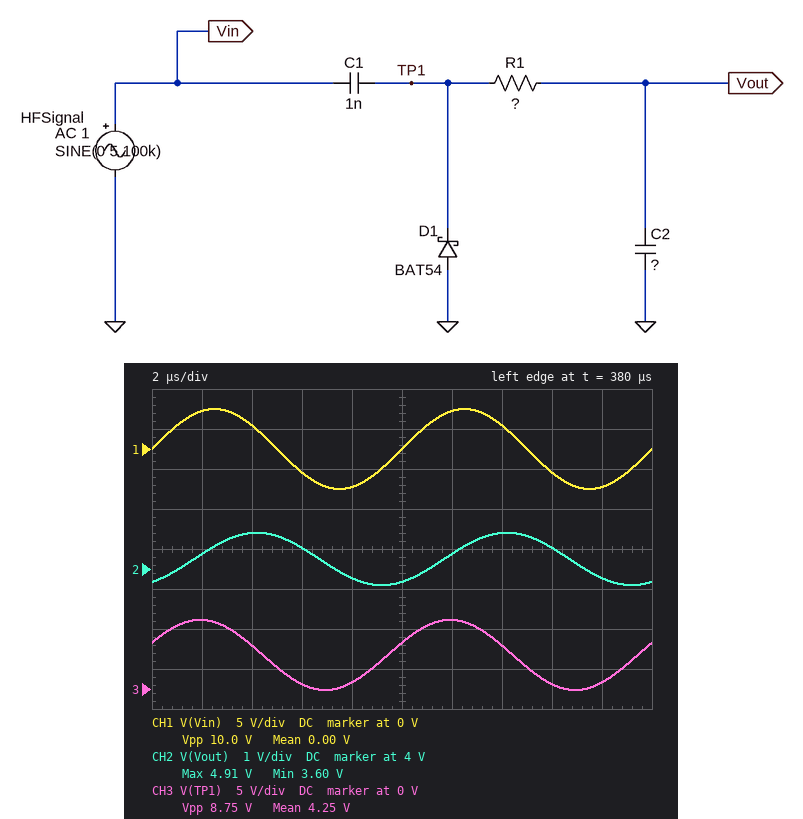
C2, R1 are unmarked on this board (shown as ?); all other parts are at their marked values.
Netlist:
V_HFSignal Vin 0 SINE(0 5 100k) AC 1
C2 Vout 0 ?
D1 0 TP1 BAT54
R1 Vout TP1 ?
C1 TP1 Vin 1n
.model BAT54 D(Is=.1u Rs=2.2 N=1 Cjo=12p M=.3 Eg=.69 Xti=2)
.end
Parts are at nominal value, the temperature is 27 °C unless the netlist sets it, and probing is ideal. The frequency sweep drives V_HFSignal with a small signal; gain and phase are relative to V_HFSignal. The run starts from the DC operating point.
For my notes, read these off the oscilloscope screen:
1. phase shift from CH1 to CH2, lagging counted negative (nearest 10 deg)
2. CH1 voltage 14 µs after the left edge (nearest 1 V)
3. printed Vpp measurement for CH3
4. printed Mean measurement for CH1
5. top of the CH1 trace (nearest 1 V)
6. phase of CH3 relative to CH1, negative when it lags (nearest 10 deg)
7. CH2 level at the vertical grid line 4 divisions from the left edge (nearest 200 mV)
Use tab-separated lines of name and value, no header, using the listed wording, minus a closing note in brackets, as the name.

phase shift from CH1 to CH2, lagging counted negative	-60 deg
CH1 voltage 14 µs after the left edge	3 V
printed Vpp measurement for CH3	8.75 V
printed Mean measurement for CH1	0.00 V
top of the CH1 trace	5 V
phase of CH3 relative to CH1, negative when it lags	20 deg
CH2 level at the vertical grid line 4 divisions from the left edge	3.8 V
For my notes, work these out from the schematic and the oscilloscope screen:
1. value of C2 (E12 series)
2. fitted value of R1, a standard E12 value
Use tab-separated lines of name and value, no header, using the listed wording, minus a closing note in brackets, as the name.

value of C2	2.7 nF
fitted value of R1, a standard E12 value	3.9 kΩ
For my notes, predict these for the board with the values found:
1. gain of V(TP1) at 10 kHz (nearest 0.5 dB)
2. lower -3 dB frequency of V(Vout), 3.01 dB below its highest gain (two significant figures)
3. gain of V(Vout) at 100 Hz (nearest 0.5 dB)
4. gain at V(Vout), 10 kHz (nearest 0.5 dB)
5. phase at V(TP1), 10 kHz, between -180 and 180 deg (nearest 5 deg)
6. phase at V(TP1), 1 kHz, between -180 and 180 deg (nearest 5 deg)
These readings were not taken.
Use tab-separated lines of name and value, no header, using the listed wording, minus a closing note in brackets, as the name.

gain of V(TP1) at 10 kHz	-10.0 dB
lower -3 dB frequency of V(Vout), 3.01 dB below its highest gain	160 Hz
gain of V(Vout) at 100 Hz	-17.0 dB
gain at V(Vout), 10 kHz	-11.5 dB
phase at V(TP1), 10 kHz, between -180 and 180 deg	25 deg
phase at V(TP1), 1 kHz, between -180 and 180 deg	10 deg
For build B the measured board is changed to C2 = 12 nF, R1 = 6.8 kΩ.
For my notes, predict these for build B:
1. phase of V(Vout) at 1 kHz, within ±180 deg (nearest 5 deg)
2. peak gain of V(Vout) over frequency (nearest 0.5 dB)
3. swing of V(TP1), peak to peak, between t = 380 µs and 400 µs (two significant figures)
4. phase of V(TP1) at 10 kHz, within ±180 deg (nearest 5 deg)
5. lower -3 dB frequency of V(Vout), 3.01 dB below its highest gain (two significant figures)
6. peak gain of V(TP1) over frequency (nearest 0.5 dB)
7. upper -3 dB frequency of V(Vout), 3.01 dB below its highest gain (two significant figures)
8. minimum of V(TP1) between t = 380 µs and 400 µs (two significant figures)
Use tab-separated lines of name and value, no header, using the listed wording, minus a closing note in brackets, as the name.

phase of V(Vout) at 1 kHz, within ±180 deg	0 deg
peak gain of V(Vout) over frequency	-22.5 dB
swing of V(TP1), peak to peak, between t = 380 µs and 400 µs	9.5 V
phase of V(TP1) at 10 kHz, within ±180 deg	60 deg
lower -3 dB frequency of V(Vout), 3.01 dB below its highest gain	46 Hz
peak gain of V(TP1) over frequency	0 dB
upper -3 dB frequency of V(Vout), 3.01 dB below its highest gain	26 kHz
minimum of V(TP1) between t = 380 µs and 400 µs	-230 mV
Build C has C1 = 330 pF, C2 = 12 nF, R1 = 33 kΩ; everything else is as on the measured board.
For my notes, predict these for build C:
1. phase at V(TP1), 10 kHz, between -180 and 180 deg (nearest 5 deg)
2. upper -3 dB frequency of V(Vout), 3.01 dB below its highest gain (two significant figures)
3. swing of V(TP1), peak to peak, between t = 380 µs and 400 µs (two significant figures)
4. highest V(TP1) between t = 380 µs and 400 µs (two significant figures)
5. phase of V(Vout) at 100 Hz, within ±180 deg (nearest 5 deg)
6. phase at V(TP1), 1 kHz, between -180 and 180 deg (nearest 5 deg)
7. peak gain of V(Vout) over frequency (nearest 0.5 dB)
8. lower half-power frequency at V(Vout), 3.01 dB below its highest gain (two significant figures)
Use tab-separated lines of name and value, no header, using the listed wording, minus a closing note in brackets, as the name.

phase at V(TP1), 10 kHz, between -180 and 180 deg	55 deg
upper -3 dB frequency of V(Vout), 3.01 dB below its highest gain	16 kHz
swing of V(TP1), peak to peak, between t = 380 µs and 400 µs	8.9 V
highest V(TP1) between t = 380 µs and 400 µs	8.7 V
phase of V(Vout) at 100 Hz, within ±180 deg	25 deg
phase at V(TP1), 1 kHz, between -180 and 180 deg	65 deg
peak gain of V(Vout) over frequency	-32.5 dB
lower half-power frequency at V(Vout), 3.01 dB below its highest gain	44 Hz
